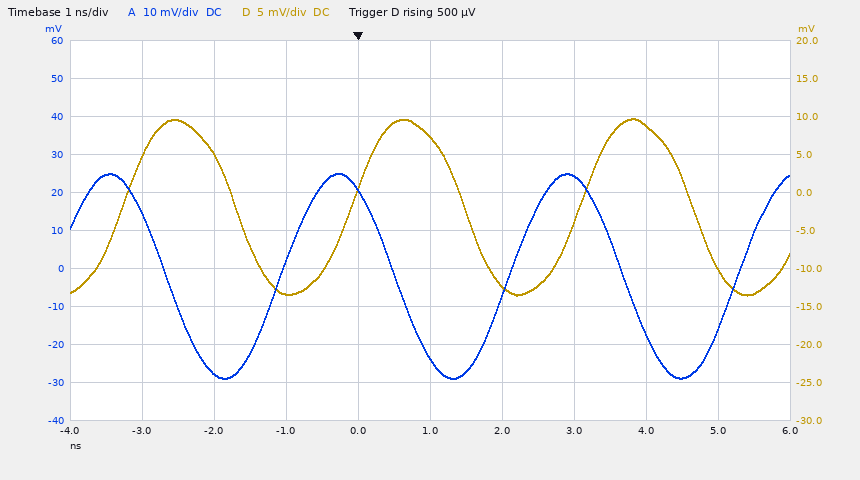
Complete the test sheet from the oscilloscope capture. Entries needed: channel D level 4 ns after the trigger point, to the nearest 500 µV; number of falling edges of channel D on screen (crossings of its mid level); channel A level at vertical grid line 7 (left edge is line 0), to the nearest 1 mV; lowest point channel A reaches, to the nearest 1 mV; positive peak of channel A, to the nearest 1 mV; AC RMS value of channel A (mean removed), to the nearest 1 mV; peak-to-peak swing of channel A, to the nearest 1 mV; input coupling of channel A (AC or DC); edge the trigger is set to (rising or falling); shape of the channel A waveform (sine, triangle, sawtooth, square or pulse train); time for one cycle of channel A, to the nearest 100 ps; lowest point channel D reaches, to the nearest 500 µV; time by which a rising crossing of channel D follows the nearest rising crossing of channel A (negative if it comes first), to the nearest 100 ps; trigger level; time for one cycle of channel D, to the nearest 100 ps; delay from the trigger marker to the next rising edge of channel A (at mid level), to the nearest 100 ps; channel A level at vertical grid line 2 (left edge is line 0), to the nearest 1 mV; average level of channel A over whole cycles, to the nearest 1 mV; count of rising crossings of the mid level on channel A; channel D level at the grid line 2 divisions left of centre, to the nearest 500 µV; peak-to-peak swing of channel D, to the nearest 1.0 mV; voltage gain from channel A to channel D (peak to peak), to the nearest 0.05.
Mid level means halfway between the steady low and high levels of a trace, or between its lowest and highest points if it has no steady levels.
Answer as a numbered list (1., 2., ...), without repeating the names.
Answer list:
1. 9.0 mV
2. 3
3. 24 mV
4. -29 mV
5. 25 mV
6. 19 mV
7. 54 mV
8. DC
9. rising
10. sine
11. 3.2 ns
12. -13.5 mV
13. +1.0 ns
14. 500 µV
15. 3.2 ns
16. 2.1 ns
17. -28 mV
18. -2 mV
19. 3
20. -13.5 mV
21. 23.0 mV
22. 0.45
